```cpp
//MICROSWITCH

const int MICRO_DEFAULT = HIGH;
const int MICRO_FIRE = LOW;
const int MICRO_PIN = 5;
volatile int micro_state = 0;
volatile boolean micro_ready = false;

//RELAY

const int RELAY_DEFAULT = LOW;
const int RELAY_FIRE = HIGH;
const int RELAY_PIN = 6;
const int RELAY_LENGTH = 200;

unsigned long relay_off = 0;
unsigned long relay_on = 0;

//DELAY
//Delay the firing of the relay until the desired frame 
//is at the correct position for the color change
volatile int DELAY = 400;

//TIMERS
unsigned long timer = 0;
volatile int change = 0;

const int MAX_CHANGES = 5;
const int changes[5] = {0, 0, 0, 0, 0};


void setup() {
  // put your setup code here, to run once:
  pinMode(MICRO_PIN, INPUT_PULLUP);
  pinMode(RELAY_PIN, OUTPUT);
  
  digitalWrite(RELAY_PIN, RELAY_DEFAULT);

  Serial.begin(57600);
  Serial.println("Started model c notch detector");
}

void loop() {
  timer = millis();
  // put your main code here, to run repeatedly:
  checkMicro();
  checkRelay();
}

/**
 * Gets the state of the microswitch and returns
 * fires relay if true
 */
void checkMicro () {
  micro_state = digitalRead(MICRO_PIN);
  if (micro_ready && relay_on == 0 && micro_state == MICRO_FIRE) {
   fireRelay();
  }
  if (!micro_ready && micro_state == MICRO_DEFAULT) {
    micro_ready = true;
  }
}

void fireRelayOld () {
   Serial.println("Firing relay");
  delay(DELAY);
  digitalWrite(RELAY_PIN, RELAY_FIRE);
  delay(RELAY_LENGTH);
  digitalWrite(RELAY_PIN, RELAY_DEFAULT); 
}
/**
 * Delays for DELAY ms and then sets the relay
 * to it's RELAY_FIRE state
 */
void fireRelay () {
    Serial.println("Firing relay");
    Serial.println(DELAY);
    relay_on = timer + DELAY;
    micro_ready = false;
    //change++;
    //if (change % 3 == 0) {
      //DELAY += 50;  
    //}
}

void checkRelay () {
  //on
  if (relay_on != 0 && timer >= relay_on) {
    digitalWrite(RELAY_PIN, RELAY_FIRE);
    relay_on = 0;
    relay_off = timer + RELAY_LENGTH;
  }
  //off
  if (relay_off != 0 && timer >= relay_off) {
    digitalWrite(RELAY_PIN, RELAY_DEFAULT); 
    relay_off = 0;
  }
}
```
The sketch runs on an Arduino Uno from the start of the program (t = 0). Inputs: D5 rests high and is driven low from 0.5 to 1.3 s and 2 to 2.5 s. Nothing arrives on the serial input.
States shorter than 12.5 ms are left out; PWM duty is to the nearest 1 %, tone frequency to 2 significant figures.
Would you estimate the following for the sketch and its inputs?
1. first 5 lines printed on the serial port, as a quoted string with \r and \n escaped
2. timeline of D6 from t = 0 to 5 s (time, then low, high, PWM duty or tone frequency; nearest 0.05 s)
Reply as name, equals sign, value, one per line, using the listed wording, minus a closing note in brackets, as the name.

first 5 lines printed on the serial port, as a quoted string with \r and \n escaped = "Started model c notch detector\r\nFiring relay\r\n400\r\nFiring relay\r\n400\r\n"
timeline of D6 from t = 0 to 5 s = 0 s low; 0.9 s high; 1.1 s low; 2.4 s high; 2.6 s low
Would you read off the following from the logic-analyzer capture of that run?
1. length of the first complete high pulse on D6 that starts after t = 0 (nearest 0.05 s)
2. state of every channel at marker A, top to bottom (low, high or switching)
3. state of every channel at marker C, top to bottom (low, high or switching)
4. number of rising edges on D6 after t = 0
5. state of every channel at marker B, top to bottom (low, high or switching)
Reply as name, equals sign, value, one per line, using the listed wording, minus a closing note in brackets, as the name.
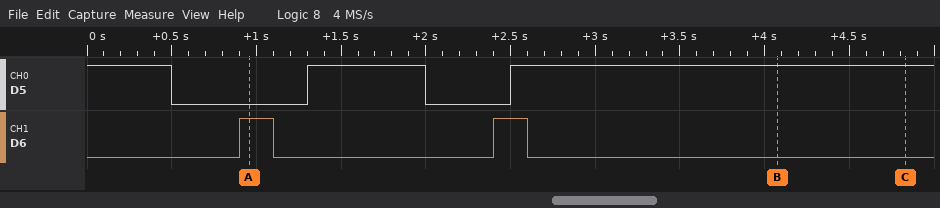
length of the first complete high pulse on D6 that starts after t = 0 = 0.20 s
state of every channel at marker A, top to bottom = D5 low, D6 high
state of every channel at marker C, top to bottom = D5 high, D6 low
number of rising edges on D6 after t = 0 = 2
state of every channel at marker B, top to bottom = D5 high, D6 low
